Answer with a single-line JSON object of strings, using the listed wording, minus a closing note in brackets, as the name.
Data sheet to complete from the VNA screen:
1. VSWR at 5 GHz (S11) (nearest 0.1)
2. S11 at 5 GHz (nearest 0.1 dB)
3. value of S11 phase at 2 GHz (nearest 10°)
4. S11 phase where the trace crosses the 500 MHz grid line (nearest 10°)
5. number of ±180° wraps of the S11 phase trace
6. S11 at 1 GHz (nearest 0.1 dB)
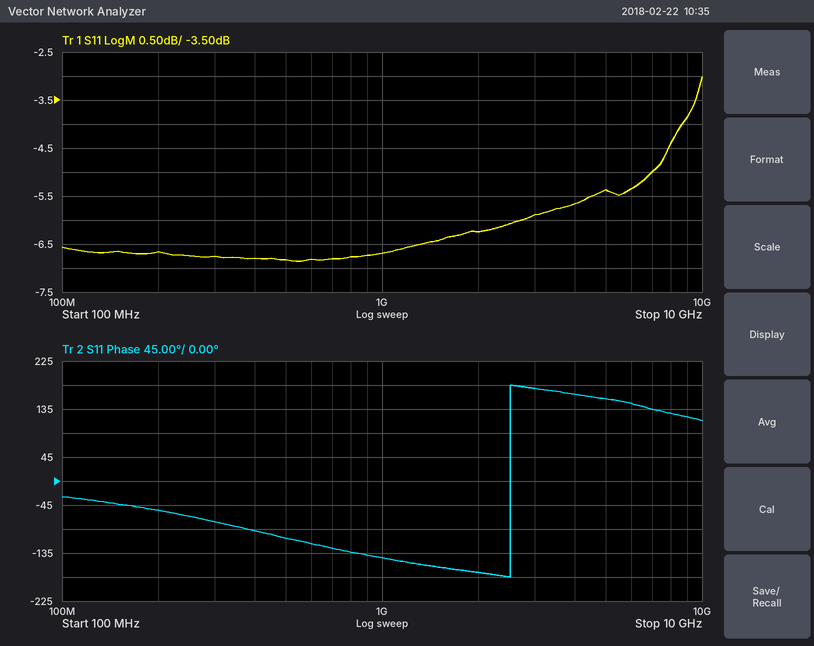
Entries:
{"VSWR at 5 GHz (S11)": "3.3", "S11 at 5 GHz": "-5.4 dB", "value of S11 phase at 2 GHz": "-170°", "S11 phase where the trace crosses the 500 MHz grid line": "-110°", "number of ±180° wraps of the S11 phase trace": "1", "S11 at 1 GHz": "-6.7 dB"}
